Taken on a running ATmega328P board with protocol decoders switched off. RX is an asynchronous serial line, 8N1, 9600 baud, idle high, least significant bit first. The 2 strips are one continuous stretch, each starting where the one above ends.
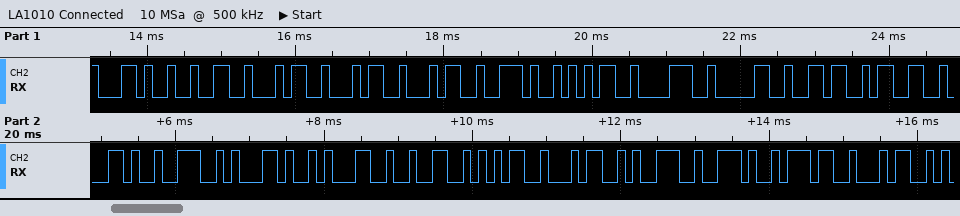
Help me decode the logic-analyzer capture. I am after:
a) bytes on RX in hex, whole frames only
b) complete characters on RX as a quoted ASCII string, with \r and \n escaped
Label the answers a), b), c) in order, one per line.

a) 2C 32 34 34 34 2E 35 38 30 36 33 2C 4E 2C 31 32 35 34 39 2E 37 34
b) ",2444.58063,N,12549.74"
